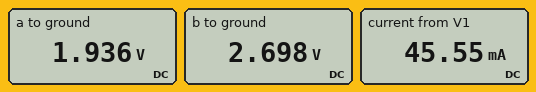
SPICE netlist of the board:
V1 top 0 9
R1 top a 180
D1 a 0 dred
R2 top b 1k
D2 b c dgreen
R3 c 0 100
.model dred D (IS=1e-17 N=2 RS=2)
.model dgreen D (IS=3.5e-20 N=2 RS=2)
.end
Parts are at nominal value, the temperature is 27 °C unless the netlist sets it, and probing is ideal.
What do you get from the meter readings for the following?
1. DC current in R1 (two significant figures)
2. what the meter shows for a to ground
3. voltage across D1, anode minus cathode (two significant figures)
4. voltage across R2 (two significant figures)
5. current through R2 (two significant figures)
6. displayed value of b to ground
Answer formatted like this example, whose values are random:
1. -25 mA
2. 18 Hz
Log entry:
1. 39 mA
2. 1.936 V
3. 1.9 V
4. 6.3 V
5. 6.3 mA
6. 2.698 V
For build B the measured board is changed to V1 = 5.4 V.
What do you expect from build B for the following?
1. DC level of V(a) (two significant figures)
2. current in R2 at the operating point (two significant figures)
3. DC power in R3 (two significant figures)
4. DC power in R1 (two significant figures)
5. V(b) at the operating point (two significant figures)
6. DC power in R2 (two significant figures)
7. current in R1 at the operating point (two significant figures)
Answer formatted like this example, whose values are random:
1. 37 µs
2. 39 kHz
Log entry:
1. 1.9 V
2. 3.1 mA
3. 940 µW
4. 70 mW
5. 2.3 V
6. 9.4 mW
7. 20 mA
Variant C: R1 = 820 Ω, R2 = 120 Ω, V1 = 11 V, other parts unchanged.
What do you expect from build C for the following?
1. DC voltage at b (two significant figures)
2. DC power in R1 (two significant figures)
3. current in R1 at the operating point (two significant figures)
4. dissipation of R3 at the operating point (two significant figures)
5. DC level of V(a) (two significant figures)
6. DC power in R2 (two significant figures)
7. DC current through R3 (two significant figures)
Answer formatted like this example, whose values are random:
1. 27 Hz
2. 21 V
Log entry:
1. 6.2 V
2. 100 mW
3. 11 mA
4. 160 mW
5. 1.8 V
6. 190 mW
7. 40 mA
